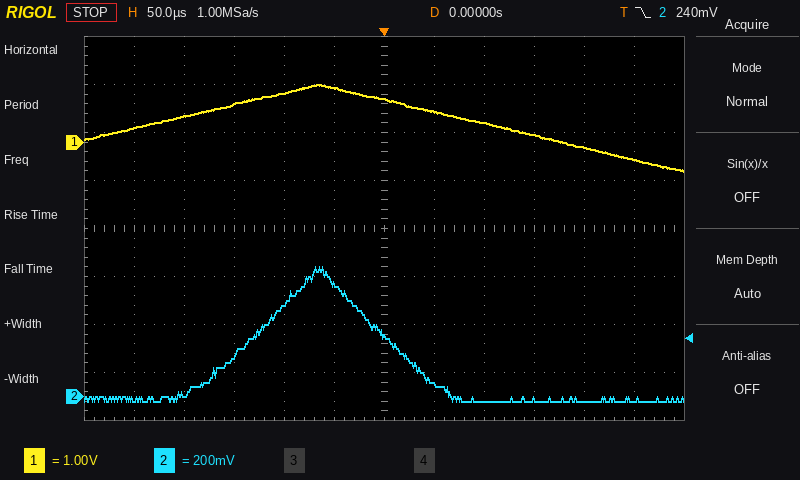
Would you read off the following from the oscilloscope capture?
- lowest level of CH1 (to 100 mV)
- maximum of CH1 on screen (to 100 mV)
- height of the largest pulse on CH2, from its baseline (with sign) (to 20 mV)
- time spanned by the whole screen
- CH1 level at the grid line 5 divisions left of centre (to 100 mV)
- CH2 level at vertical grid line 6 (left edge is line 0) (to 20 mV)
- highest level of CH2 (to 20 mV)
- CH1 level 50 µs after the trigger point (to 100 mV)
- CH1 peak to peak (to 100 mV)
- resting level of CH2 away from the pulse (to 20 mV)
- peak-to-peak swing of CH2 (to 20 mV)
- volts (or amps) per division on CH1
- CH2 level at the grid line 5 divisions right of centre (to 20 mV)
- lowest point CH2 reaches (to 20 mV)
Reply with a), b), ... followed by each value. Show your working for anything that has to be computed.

a) -600 mV
b) 1.2 V
c) 540 mV − (-20 mV) = +560 mV
d) 600 µs
e) 300 mV
f) 260 mV
g) 540 mV
h) 600 mV
i) 1.2 V − (-600 mV) = 1.8 V
j) -20 mV
k) 540 mV − (-20 mV) = 560 mV
l) 1 V
m) -20 mV
n) -20 mV
